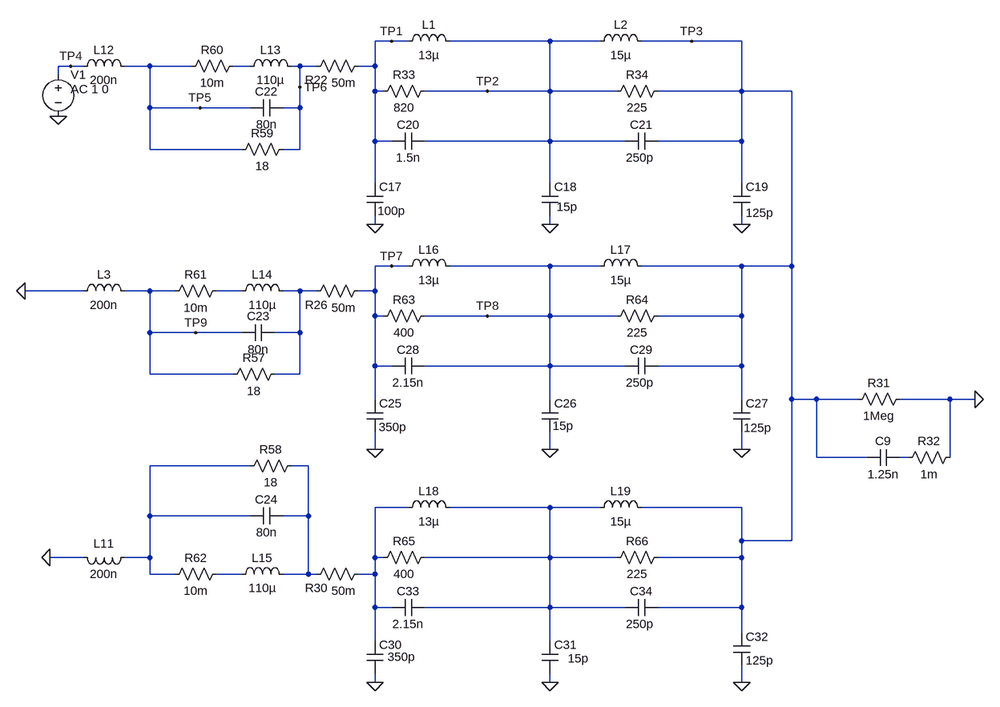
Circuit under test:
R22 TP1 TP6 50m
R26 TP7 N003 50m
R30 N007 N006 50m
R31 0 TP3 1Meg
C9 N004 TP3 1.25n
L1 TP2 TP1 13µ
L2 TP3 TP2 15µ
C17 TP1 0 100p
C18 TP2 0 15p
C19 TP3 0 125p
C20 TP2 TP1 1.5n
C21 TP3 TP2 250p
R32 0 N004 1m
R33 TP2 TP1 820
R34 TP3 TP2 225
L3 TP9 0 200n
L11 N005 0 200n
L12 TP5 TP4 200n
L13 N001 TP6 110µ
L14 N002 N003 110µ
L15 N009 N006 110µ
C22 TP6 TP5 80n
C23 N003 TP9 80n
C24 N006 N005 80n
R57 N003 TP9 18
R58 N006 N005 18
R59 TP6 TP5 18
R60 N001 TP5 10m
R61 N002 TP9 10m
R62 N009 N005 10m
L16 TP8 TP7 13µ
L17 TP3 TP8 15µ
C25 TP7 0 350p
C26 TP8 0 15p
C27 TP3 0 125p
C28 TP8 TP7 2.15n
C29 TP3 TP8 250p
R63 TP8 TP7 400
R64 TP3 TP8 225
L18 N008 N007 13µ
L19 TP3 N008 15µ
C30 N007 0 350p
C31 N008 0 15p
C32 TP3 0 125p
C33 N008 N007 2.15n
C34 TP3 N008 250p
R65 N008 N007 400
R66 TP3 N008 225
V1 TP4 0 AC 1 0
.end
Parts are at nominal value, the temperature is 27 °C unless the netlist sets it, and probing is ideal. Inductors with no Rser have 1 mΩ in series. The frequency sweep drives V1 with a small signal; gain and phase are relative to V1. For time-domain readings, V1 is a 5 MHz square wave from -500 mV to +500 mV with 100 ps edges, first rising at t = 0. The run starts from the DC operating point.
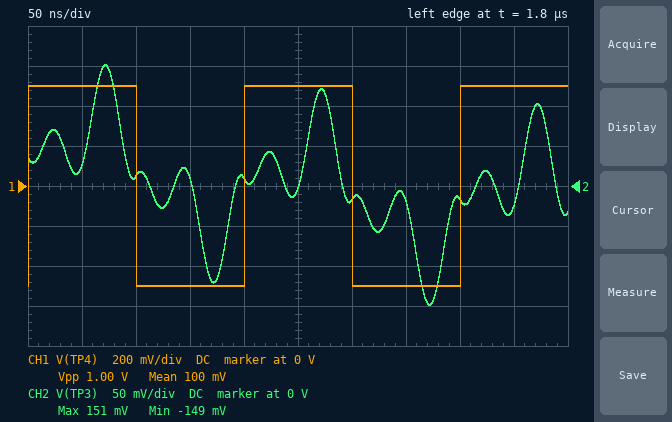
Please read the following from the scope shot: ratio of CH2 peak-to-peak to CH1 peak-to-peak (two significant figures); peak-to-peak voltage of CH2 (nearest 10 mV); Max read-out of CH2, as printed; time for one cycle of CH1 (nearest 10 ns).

0.30
300 mV
151 mV
200 ns
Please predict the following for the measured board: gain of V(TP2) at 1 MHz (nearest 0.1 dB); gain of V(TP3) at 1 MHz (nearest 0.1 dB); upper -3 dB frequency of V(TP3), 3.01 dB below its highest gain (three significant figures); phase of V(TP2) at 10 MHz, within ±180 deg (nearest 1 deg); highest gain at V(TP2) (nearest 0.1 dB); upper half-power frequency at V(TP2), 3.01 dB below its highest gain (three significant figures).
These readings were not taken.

-13.5 dB
-13.6 dB
21.2 MHz
-1 deg
22.0 dB
21.2 MHz
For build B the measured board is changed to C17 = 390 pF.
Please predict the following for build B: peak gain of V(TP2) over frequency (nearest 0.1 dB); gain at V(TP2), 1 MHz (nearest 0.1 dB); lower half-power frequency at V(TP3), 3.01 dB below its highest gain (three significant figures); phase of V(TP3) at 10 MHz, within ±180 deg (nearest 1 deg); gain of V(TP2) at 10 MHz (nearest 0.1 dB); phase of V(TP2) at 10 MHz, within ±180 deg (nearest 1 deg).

21.8 dB
-13.5 dB
15.2 MHz
-13 deg
4.0 dB
-2 deg
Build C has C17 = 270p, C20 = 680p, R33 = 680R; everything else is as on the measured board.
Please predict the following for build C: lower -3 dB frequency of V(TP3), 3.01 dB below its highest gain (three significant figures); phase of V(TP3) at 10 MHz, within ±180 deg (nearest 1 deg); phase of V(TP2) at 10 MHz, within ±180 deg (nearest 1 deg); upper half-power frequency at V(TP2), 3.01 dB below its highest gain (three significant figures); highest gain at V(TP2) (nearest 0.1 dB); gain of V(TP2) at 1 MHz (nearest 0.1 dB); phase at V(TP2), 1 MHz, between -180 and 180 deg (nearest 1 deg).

16.6 MHz
-10 deg
1 deg
17.4 MHz
24.7 dB
-6.6 dB
-42 deg
